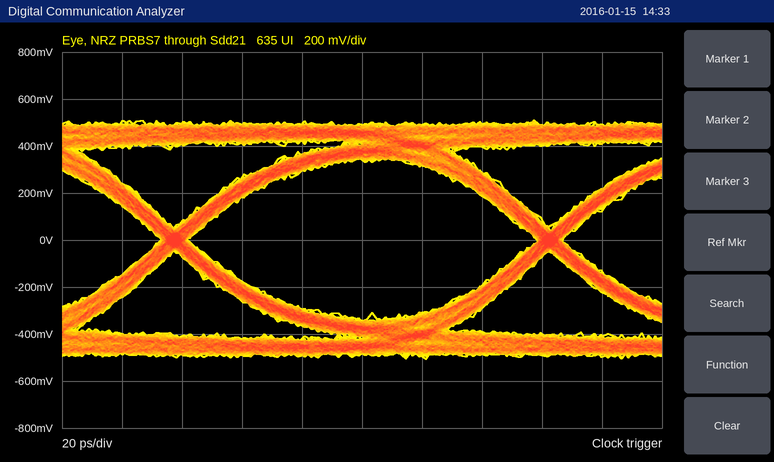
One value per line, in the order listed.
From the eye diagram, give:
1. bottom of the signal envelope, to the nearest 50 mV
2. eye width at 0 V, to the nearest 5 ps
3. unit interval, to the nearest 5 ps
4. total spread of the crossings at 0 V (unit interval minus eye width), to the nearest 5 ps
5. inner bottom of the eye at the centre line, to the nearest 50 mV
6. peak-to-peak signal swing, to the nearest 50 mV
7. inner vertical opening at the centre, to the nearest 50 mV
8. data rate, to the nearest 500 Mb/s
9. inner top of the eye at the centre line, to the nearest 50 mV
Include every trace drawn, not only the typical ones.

-500 mV
115 ps
125 ps
10 ps
-350 mV
1.00 V
700 mV
8.0 Gb/s
350 mV
